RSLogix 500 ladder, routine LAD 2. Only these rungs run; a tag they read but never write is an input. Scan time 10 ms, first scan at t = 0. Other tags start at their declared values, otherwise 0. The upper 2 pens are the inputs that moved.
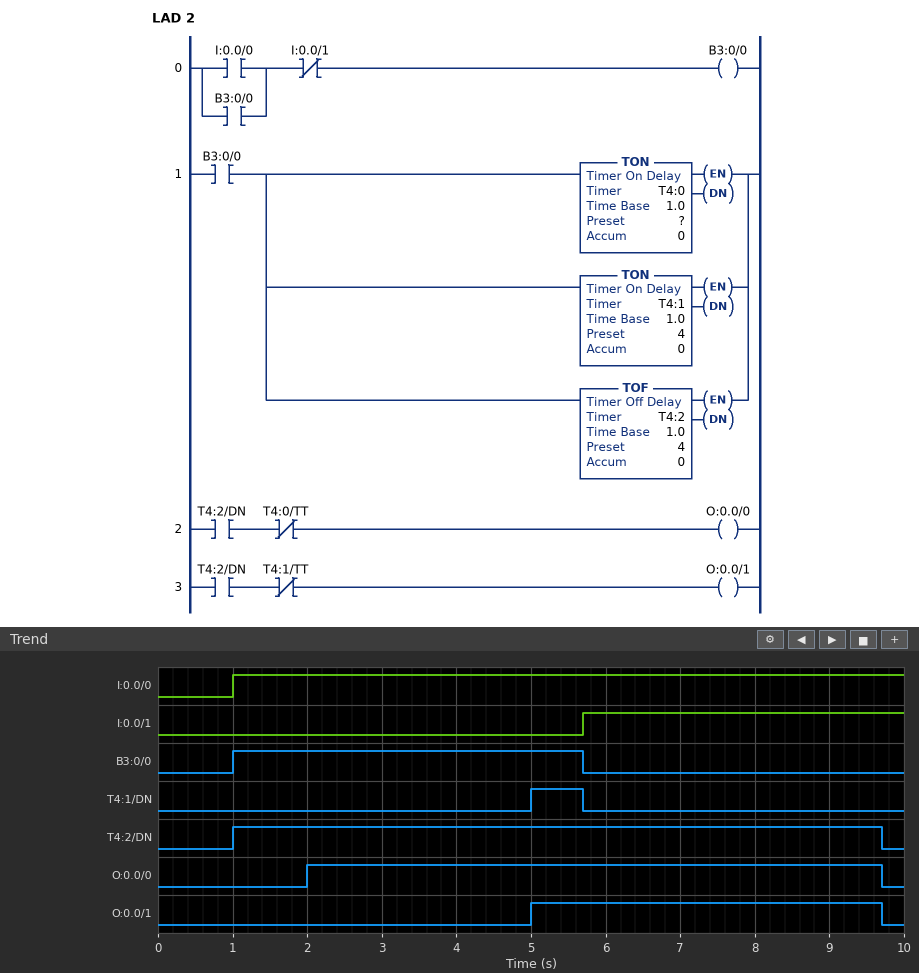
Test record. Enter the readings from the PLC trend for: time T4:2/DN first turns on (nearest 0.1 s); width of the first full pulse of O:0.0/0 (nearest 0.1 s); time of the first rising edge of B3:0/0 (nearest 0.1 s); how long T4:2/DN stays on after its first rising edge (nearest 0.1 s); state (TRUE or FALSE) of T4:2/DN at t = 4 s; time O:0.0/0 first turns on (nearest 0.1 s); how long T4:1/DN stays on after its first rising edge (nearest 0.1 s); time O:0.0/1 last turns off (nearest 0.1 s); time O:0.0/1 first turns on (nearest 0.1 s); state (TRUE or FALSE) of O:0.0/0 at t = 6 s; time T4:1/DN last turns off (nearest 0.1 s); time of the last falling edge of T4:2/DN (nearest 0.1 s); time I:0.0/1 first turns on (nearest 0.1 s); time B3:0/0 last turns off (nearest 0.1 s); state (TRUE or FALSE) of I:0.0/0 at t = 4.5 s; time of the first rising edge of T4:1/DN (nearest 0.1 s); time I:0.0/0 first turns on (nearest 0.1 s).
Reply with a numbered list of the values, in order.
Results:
1. 1.0 s
2. 7.7 s
3. 1.0 s
4. 8.7 s
5. TRUE
6. 2.0 s
7. 0.7 s
8. 9.7 s
9. 5.0 s
10. TRUE
11. 5.7 s
12. 9.7 s
13. 5.7 s
14. 5.7 s
15. TRUE
16. 5.0 s
17. 1.0 s
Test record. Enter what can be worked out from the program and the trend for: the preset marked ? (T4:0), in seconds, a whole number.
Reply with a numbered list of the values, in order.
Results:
1. 1 s
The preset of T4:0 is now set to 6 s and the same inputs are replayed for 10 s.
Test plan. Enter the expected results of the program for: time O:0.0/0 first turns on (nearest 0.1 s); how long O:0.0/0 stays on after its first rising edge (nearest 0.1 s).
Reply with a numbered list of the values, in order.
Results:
1. 5.7 s
2. 4.0 s
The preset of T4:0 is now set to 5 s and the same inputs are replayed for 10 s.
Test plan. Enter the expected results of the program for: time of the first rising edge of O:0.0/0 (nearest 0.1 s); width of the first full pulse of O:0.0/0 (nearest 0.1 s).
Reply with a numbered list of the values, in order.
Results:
1. 5.7 s
2. 4.0 s
